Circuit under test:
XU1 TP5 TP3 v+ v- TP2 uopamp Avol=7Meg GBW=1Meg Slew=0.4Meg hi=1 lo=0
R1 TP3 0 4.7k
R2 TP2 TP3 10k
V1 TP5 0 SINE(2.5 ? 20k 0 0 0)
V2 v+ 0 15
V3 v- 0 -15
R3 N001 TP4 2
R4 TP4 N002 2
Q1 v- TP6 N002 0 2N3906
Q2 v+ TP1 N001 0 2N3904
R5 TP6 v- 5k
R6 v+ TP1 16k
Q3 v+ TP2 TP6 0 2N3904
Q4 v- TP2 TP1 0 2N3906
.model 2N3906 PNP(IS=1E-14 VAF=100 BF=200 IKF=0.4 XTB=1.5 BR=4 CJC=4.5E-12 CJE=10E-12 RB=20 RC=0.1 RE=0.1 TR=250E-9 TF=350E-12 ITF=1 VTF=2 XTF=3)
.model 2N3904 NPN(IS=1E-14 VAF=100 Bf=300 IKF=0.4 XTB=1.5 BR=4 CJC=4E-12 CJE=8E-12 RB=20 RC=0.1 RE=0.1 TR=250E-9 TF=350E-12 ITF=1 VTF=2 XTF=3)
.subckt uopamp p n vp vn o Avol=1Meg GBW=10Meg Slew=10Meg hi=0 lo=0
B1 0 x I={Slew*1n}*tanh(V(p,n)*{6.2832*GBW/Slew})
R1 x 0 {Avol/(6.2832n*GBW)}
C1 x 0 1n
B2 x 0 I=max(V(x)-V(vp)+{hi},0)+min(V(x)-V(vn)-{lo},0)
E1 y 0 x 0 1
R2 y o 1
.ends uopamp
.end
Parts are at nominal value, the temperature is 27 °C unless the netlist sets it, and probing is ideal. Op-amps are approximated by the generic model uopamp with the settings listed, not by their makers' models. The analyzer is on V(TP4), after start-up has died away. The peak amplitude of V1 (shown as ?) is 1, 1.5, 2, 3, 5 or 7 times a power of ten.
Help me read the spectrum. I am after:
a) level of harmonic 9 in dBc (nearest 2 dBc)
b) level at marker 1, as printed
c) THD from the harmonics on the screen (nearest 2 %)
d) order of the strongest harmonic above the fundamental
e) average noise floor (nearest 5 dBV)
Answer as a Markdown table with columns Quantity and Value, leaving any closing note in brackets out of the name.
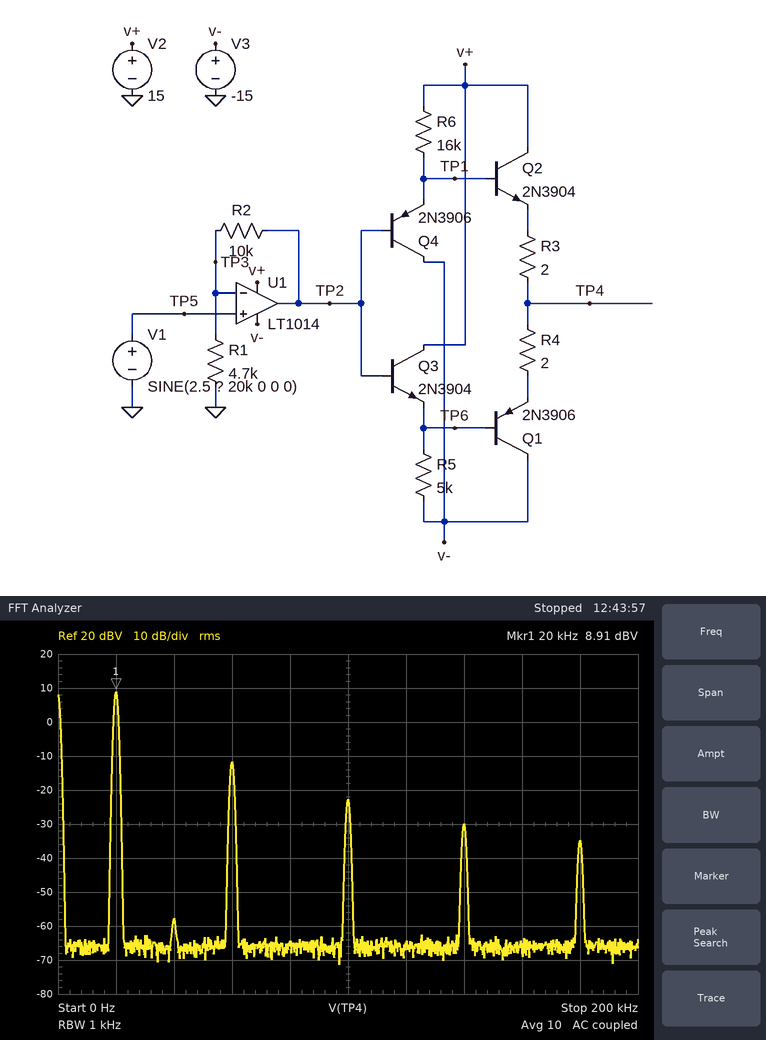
| Quantity | Value |
|---|---|
| level of harmonic 9 in dBc | -44 dBc |
| level at marker 1, as printed | 8.91 dBV |
| THD from the harmonics on the screen | 10 % |
| order of the strongest harmonic above the fundamental | 3 |
| average noise floor | -65 dBV |
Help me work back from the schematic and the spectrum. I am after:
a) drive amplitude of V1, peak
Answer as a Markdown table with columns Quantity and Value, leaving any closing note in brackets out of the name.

| Quantity | Value |
|---|---|
| drive amplitude of V1, peak | 1.5 V |
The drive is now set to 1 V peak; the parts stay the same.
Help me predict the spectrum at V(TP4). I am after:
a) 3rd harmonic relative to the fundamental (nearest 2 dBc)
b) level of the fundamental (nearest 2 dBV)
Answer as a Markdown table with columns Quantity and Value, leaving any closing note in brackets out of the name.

| Quantity | Value |
|---|---|
| 3rd harmonic relative to the fundamental | -36 dBc |
| level of the fundamental | 6 dBV |
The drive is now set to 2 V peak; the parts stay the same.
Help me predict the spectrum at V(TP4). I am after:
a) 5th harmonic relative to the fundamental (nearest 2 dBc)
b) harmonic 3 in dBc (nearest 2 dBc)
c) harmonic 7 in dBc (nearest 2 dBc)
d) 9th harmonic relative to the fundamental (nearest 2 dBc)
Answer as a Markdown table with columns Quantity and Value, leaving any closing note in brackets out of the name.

| Quantity | Value |
|---|---|
| 5th harmonic relative to the fundamental | -28 dBc |
| harmonic 3 in dBc | -20 dBc |
| harmonic 7 in dBc | -34 dBc |
| 9th harmonic relative to the fundamental | -40 dBc |
